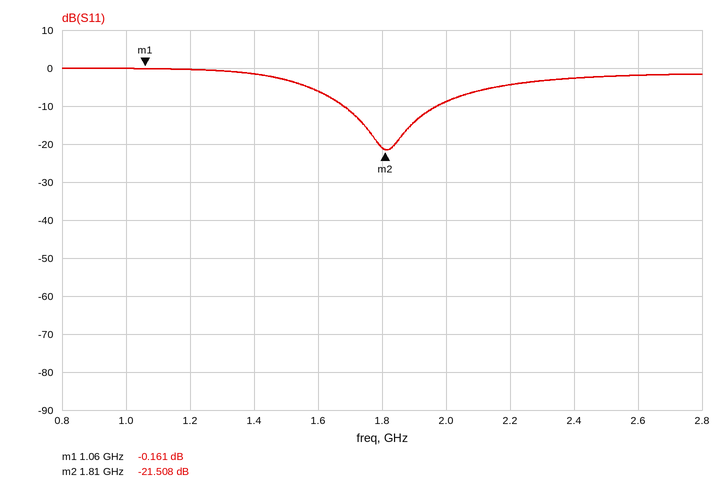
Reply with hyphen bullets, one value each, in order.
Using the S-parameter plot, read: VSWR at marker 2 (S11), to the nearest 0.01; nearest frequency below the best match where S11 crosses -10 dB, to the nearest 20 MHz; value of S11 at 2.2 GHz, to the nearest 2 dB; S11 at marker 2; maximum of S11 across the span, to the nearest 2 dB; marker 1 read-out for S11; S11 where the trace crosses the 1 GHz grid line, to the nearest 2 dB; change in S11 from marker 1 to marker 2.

- 1.18
- 1.68 GHz
- -4 dB
- -21.508 dB
- 0 dB
- -0.161 dB
- 0 dB
- -21.347 dB
